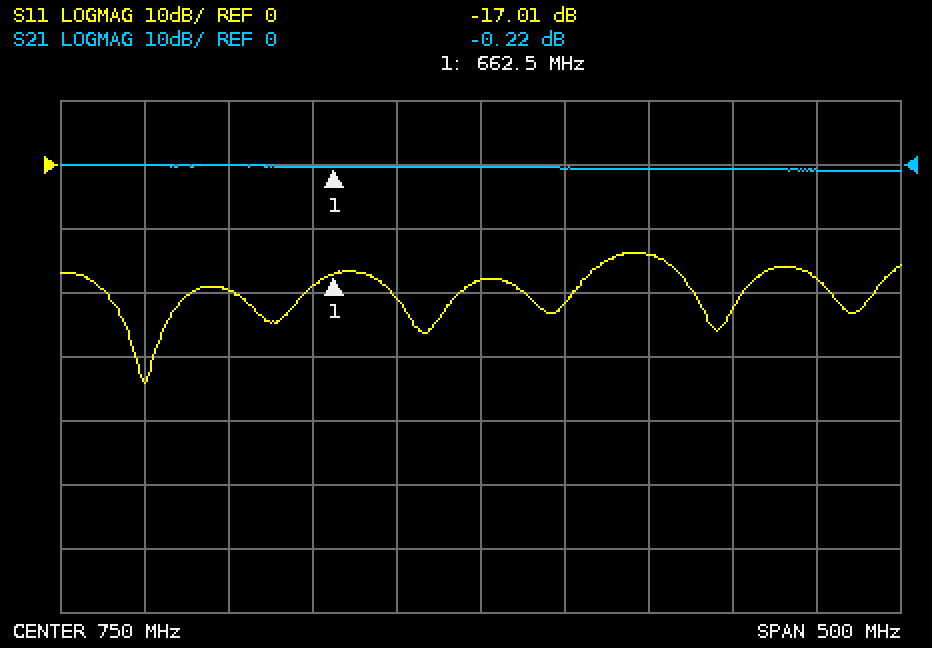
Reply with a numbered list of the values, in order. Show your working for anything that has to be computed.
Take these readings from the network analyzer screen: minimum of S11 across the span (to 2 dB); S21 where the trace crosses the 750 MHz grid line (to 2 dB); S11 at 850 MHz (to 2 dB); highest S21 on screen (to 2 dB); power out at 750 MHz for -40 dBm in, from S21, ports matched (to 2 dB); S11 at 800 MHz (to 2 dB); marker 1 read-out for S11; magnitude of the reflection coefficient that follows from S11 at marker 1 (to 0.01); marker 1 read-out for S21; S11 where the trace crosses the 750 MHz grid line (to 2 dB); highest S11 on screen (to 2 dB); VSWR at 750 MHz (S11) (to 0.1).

1. -34 dB
2. 0 dB
3. -14 dB
4. 0 dB
5. -40 dBm + (0 dB) = -40 dBm
6. -22 dB
7. -17.01 dB
8. 10^(-17.01/20) ≈ 0.14
9. -0.22 dB
10. -18 dB
11. -14 dB
12. |Γ| = 10^(-18/20) = 0.1259; VSWR = (1 + 0.1259)/(1 − 0.1259) ≈ 1.3
